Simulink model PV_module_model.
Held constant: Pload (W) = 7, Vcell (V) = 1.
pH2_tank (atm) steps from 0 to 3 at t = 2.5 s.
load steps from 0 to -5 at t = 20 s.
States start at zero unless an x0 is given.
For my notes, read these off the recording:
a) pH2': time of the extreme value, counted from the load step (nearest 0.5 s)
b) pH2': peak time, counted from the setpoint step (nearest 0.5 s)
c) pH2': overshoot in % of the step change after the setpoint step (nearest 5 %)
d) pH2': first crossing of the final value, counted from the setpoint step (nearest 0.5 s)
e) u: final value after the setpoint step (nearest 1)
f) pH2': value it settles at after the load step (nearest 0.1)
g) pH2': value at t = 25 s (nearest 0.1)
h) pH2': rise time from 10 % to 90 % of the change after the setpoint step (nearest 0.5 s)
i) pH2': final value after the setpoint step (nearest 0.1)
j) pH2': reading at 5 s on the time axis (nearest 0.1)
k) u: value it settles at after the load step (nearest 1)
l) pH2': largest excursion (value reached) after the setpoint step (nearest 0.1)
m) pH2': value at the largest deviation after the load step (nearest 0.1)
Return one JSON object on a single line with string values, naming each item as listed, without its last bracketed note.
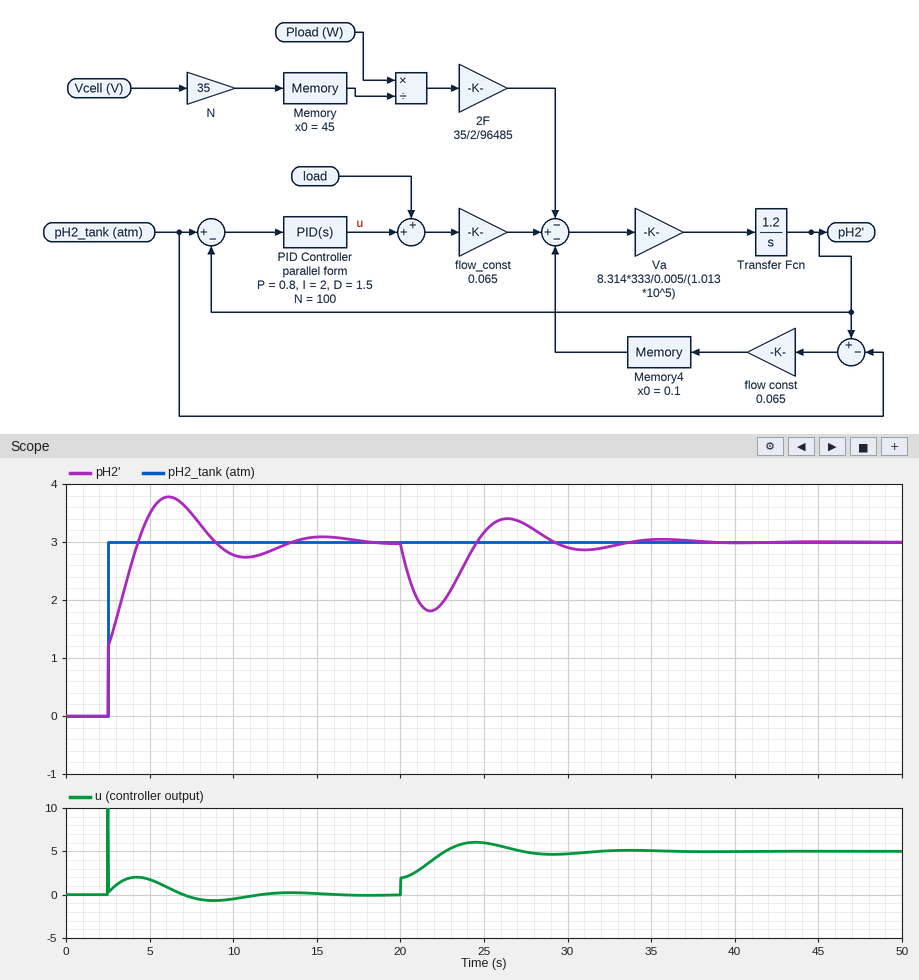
{"pH2': time of the extreme value, counted from the load step": "2.0 s", "pH2': peak time, counted from the setpoint step": "3.5 s", "pH2': overshoot in % of the step change after the setpoint step": "25 %", "pH2': first crossing of the final value, counted from the setpoint step": "2.0 s", "u: final value after the setpoint step": "0", "pH2': value it settles at after the load step": "3.0", "pH2': value at t = 25 s": "3.2", "pH2': rise time from 10 % to 90 % of the change after the setpoint step": "1.5 s", "pH2': final value after the setpoint step": "3.0", "pH2': reading at 5 s on the time axis": "3.5", "u: value it settles at after the load step": "5", "pH2': largest excursion (value reached) after the setpoint step": "3.8", "pH2': value at the largest deviation after the load step": "1.8"}
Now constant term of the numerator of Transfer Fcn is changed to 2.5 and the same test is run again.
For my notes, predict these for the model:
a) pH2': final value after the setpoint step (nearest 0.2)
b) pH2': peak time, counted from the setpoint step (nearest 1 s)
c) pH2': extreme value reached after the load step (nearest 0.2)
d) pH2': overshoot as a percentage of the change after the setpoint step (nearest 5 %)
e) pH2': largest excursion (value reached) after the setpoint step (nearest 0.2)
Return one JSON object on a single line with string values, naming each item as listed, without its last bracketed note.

{"pH2': final value after the setpoint step": "3.0", "pH2': peak time, counted from the setpoint step": "3 s", "pH2': extreme value reached after the load step": "1.6", "pH2': overshoot as a percentage of the change after the setpoint step": "15 %", "pH2': largest excursion (value reached) after the setpoint step": "3.4"}
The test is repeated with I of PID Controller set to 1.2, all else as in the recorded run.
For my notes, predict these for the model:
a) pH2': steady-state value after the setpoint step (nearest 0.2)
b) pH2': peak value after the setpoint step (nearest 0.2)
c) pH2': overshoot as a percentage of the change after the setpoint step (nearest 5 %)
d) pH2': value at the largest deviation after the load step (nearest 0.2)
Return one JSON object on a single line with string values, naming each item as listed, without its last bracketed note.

{"pH2': steady-state value after the setpoint step": "3.0", "pH2': peak value after the setpoint step": "3.6", "pH2': overshoot as a percentage of the change after the setpoint step": "20 %", "pH2': value at the largest deviation after the load step": "1.6"}
